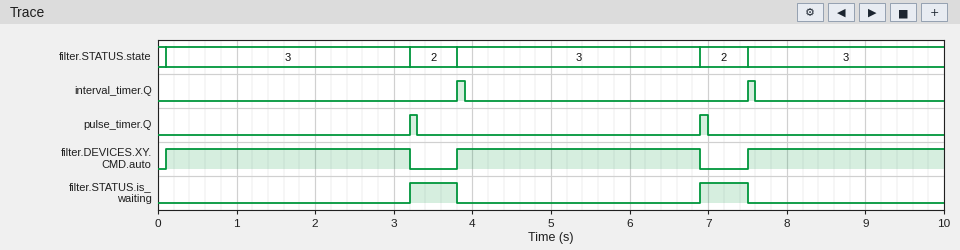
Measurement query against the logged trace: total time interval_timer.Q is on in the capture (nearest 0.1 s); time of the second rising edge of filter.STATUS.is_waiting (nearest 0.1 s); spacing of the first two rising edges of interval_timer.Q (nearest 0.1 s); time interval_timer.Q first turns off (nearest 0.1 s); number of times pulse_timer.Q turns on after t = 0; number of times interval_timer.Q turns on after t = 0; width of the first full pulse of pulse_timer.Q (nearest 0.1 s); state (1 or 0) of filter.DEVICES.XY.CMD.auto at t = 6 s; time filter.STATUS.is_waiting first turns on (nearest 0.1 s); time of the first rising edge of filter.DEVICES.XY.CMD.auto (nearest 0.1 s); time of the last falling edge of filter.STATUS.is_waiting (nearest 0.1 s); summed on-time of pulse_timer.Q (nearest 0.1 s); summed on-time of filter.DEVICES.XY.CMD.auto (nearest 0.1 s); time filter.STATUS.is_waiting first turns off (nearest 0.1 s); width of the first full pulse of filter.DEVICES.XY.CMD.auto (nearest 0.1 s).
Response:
0.2 s
6.9 s
3.7 s
3.9 s
2
2
0.1 s
1
3.2 s
0.1 s
7.5 s
0.2 s
8.7 s
3.8 s
3.1 s
